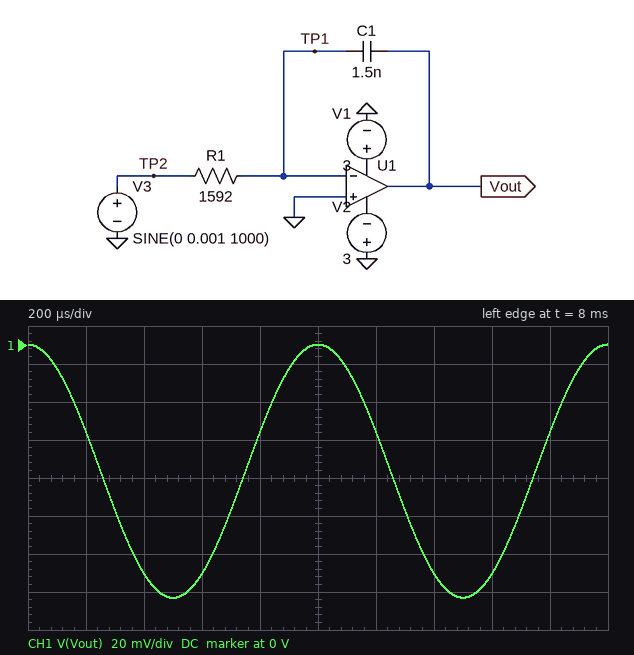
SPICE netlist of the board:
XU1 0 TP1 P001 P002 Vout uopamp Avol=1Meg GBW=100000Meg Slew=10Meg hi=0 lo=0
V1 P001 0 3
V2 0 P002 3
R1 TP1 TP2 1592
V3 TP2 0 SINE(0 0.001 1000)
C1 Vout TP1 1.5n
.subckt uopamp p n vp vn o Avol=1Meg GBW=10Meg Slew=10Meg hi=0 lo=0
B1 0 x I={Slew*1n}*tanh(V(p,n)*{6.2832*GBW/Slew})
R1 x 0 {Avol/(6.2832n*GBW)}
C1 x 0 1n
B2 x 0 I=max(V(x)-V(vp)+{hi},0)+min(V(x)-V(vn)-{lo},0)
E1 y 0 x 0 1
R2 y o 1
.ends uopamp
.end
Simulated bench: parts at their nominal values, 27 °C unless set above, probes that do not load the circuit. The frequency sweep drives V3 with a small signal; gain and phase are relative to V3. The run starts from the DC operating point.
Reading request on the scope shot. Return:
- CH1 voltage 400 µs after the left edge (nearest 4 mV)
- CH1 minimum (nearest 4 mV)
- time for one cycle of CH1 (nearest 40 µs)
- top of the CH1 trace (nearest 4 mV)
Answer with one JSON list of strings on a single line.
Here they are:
["-120 mV", "-132 mV", "1.00 ms", "0 V"]
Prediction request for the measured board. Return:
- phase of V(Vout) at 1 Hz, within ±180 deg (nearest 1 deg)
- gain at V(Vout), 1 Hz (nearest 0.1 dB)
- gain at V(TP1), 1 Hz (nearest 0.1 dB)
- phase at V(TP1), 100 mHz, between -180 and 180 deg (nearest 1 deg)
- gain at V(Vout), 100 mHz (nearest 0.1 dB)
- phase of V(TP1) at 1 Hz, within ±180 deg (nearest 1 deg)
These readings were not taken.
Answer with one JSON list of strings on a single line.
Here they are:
["94 deg", "96.5 dB", "-23.5 dB", "-56 deg", "114.9 dB", "-86 deg"]
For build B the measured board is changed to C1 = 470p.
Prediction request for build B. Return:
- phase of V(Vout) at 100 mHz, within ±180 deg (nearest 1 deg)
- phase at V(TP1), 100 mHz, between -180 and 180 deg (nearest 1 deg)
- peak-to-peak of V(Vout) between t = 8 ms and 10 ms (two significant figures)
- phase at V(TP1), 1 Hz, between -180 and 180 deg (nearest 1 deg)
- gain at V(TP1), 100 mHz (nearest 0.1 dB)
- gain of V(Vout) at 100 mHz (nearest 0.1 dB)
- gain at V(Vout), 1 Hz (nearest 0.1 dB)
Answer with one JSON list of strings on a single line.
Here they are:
["155 deg", "-25 deg", "430 mV", "-78 deg", "-0.9 dB", "119.1 dB", "106.4 dB"]
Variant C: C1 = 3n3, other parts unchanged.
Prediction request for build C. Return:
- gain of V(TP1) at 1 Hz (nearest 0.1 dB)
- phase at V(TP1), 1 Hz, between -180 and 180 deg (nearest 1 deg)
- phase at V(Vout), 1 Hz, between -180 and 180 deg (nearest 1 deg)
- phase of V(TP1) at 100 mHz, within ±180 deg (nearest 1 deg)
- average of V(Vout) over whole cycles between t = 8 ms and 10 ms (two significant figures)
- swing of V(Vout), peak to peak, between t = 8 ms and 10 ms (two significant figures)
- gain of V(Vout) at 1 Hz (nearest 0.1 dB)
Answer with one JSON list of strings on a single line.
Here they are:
["-30.4 dB", "-88 deg", "92 deg", "-73 deg", "-30 mV", "61 mV", "89.6 dB"]
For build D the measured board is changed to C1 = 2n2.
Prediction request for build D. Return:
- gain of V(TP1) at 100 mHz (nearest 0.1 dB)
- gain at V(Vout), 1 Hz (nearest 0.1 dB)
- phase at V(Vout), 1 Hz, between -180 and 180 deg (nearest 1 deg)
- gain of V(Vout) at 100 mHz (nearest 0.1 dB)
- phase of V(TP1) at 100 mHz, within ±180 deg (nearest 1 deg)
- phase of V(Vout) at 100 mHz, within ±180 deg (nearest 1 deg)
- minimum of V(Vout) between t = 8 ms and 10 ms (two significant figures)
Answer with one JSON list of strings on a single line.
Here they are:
["-7.7 dB", "93.1 dB", "93 deg", "112.3 dB", "-66 deg", "114 deg", "-91 mV"]
